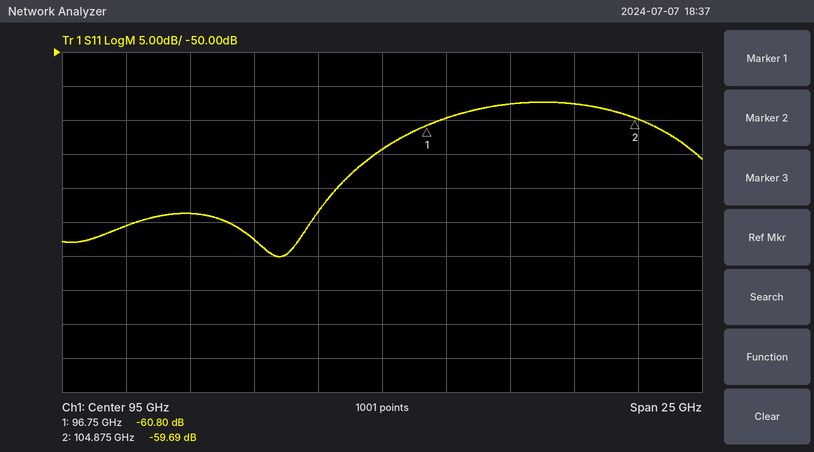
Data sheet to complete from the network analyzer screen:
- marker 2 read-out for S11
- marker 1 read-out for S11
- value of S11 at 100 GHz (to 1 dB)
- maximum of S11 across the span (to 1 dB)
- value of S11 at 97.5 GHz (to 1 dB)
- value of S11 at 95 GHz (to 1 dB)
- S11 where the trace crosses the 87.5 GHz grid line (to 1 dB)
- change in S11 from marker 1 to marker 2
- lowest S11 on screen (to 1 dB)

-59.69 dB
-60.80 dB
-58 dB
-57 dB
-60 dB
-64 dB
-74 dB
1.11 dB
-80 dB
